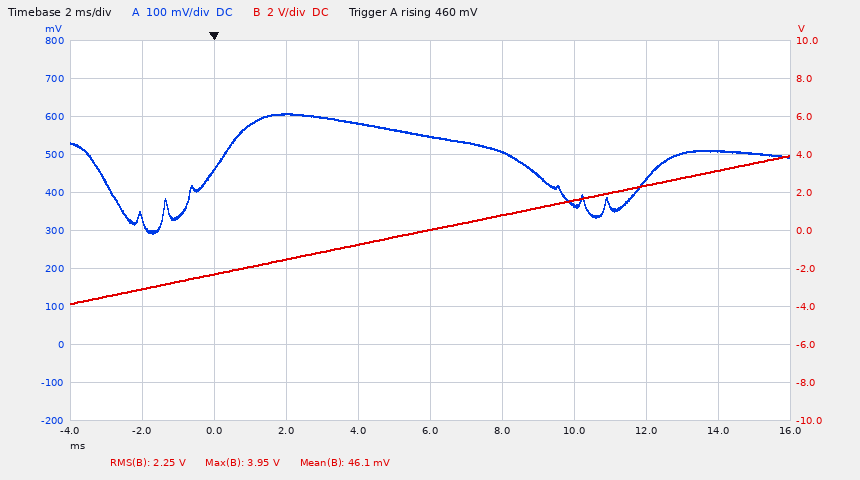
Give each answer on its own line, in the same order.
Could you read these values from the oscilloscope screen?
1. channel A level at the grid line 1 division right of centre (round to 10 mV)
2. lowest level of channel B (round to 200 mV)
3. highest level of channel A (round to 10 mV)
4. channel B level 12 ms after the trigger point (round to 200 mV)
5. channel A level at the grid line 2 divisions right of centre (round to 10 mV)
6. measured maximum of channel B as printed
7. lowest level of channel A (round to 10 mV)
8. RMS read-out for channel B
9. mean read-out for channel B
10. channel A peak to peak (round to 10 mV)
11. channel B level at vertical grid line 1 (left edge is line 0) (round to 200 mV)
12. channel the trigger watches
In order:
510 mV
-3.8 V
610 mV
2.4 V
370 mV
3.95 V
290 mV
2.25 V
46.1 mV
320 mV
-3.0 V
channel A
